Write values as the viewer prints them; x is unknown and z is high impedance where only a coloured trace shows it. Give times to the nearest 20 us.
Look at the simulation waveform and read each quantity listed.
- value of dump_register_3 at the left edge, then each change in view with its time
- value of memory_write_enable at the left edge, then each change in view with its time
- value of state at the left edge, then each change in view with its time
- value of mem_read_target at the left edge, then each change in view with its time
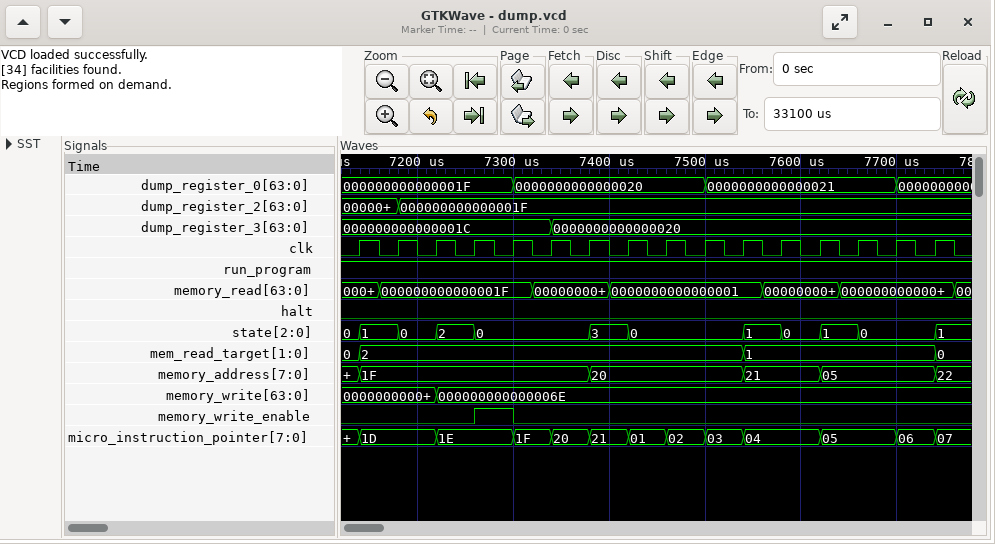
000000000000001C, 0000000000000020 at 7340 us
0, 1 at 7260 us, 0 at 7300 us
0, 1 at 7140 us, 0 at 7180 us, 2 at 7220 us, 0 at 7260 us, 3 at 7380 us, 0 at 7420 us, 1 at 7540 us, 0 at 7580 us, 1 at 7620 us, 0 at 7660 us, 1 at 7740 us
0, 2 at 7140 us, 1 at 7540 us, 0 at 7740 us
